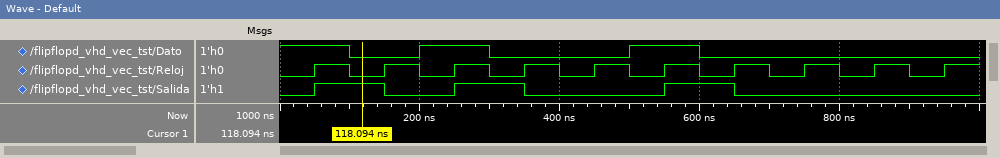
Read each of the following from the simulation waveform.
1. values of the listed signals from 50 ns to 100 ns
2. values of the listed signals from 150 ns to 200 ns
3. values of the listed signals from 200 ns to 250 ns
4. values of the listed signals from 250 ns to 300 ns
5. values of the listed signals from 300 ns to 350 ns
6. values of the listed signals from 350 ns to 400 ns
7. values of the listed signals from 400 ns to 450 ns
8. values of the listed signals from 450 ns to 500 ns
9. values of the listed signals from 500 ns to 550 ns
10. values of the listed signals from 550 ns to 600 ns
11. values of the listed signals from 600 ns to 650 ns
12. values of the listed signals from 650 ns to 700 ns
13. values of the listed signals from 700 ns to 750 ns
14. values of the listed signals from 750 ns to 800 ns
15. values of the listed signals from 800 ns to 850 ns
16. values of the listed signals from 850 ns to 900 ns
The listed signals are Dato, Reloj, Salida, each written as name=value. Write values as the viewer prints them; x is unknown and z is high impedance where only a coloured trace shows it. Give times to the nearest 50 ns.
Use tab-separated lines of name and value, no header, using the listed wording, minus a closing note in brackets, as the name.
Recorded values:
values of the listed signals from 50 ns to 100 ns	Dato=1, Reloj=1, Salida=1
values of the listed signals from 150 ns to 200 ns	Dato=0, Reloj=1, Salida=0
values of the listed signals from 200 ns to 250 ns	Dato=1, Reloj=0, Salida=0
values of the listed signals from 250 ns to 300 ns	Dato=1, Reloj=1, Salida=1
values of the listed signals from 300 ns to 350 ns	Dato=0, Reloj=0, Salida=1
values of the listed signals from 350 ns to 400 ns	Dato=0, Reloj=1, Salida=0
values of the listed signals from 400 ns to 450 ns	Dato=0, Reloj=0, Salida=0
values of the listed signals from 450 ns to 500 ns	Dato=0, Reloj=1, Salida=0
values of the listed signals from 500 ns to 550 ns	Dato=1, Reloj=0, Salida=0
values of the listed signals from 550 ns to 600 ns	Dato=1, Reloj=1, Salida=1
values of the listed signals from 600 ns to 650 ns	Dato=0, Reloj=0, Salida=1
values of the listed signals from 650 ns to 700 ns	Dato=0, Reloj=1, Salida=0
values of the listed signals from 700 ns to 750 ns	Dato=0, Reloj=0, Salida=0
values of the listed signals from 750 ns to 800 ns	Dato=0, Reloj=1, Salida=0
values of the listed signals from 800 ns to 850 ns	Dato=0, Reloj=0, Salida=0
values of the listed signals from 850 ns to 900 ns	Dato=0, Reloj=1, Salida=0
